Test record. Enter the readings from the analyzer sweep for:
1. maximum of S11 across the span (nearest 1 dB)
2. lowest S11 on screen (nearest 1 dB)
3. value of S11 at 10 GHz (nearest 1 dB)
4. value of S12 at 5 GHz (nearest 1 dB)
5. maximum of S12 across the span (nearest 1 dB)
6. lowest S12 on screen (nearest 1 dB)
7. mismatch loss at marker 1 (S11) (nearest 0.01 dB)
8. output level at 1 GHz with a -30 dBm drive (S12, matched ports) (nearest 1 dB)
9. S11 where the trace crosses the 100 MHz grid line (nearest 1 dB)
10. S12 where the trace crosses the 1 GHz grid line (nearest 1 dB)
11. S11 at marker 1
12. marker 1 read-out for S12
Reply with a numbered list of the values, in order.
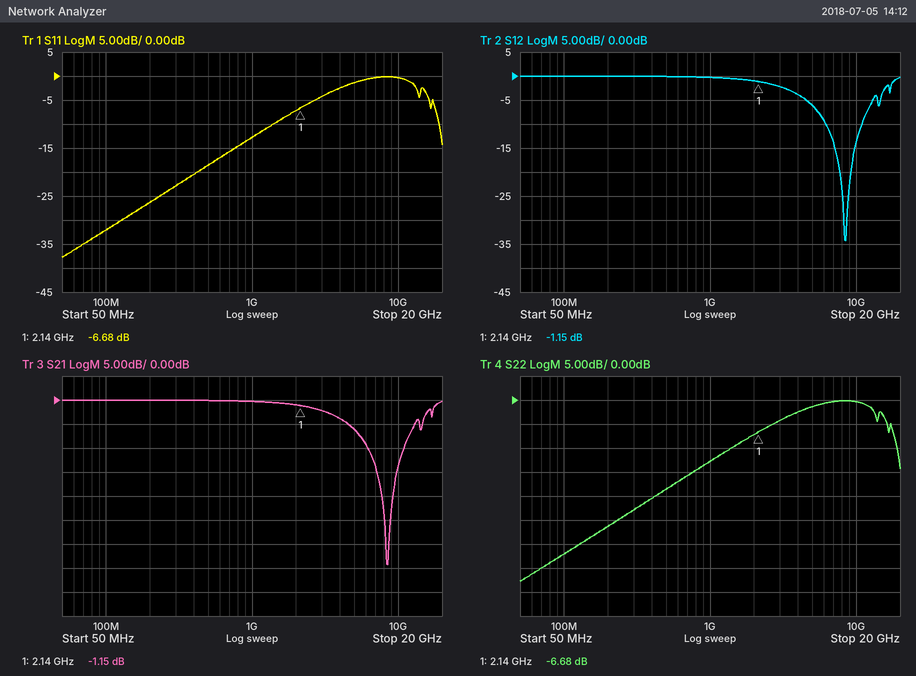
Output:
1. 0 dB
2. -38 dB
3. 0 dB
4. -6 dB
5. 0 dB
6. -34 dB
7. 1.05 dB
8. -30 dBm
9. -32 dB
10. 0 dB
11. -6.68 dB
12. -1.15 dB
